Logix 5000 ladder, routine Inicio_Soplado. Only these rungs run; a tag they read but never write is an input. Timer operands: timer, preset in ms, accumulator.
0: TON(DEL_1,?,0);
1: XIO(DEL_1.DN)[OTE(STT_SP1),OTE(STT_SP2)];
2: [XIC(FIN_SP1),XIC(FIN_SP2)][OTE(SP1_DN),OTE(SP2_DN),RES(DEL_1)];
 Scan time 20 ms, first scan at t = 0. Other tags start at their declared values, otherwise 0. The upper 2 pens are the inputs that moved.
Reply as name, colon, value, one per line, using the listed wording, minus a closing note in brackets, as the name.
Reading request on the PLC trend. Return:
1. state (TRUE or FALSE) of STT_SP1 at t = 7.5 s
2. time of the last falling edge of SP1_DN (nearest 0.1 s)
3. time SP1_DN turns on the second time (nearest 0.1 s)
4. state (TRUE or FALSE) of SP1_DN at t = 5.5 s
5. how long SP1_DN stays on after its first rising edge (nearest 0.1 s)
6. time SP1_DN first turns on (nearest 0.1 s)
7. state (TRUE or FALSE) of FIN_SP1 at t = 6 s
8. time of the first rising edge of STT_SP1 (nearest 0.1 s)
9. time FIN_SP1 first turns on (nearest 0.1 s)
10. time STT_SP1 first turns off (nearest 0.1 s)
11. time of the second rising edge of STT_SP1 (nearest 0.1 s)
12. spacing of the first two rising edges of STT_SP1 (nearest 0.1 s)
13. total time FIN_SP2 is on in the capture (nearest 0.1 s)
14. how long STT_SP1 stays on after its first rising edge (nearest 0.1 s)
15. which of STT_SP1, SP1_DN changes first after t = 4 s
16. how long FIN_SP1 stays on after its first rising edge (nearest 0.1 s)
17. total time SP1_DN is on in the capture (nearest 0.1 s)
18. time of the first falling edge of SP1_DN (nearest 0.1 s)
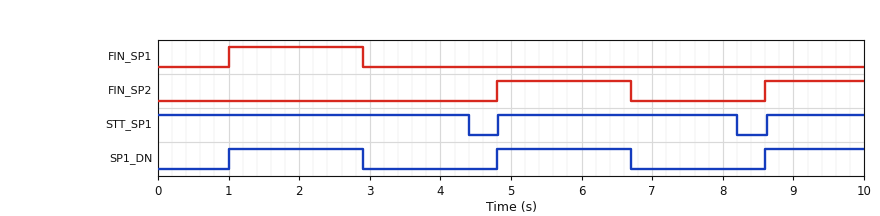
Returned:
state (TRUE or FALSE) of STT_SP1 at t = 7.5 s: TRUE
time of the last falling edge of SP1_DN: 6.7 s
time SP1_DN turns on the second time: 4.8 s
state (TRUE or FALSE) of SP1_DN at t = 5.5 s: TRUE
how long SP1_DN stays on after its first rising edge: 1.9 s
time SP1_DN first turns on: 1.0 s
state (TRUE or FALSE) of FIN_SP1 at t = 6 s: FALSE
time of the first rising edge of STT_SP1: 4.8 s
time FIN_SP1 first turns on: 1.0 s
time STT_SP1 first turns off: 4.4 s
time of the second rising edge of STT_SP1: 8.6 s
spacing of the first two rising edges of STT_SP1: 3.8 s
total time FIN_SP2 is on in the capture: 3.3 s
how long STT_SP1 stays on after its first rising edge: 3.4 s
which of STT_SP1, SP1_DN changes first after t = 4 s: STT_SP1
how long FIN_SP1 stays on after its first rising edge: 1.9 s
total time SP1_DN is on in the capture: 5.2 s
time of the first falling edge of SP1_DN: 2.9 s
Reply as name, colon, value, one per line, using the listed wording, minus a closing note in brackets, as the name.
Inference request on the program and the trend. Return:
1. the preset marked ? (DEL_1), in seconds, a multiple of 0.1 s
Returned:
the preset marked ? (DEL_1), in seconds, a multiple of 0.1 s: 1.5 s
